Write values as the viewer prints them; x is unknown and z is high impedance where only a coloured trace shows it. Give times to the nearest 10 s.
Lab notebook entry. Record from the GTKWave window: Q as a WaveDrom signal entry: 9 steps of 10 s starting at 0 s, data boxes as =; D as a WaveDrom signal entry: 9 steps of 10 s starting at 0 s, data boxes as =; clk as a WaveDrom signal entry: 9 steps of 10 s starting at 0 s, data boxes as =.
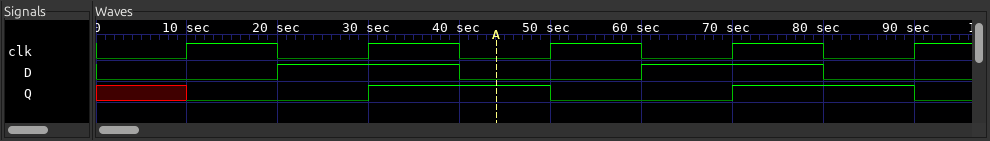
{name: 'Q', wave: 'x0.1.0.1.'}
{name: 'D', wave: '0.1.0.1.0'}
{name: 'clk', wave: '010101010'}
